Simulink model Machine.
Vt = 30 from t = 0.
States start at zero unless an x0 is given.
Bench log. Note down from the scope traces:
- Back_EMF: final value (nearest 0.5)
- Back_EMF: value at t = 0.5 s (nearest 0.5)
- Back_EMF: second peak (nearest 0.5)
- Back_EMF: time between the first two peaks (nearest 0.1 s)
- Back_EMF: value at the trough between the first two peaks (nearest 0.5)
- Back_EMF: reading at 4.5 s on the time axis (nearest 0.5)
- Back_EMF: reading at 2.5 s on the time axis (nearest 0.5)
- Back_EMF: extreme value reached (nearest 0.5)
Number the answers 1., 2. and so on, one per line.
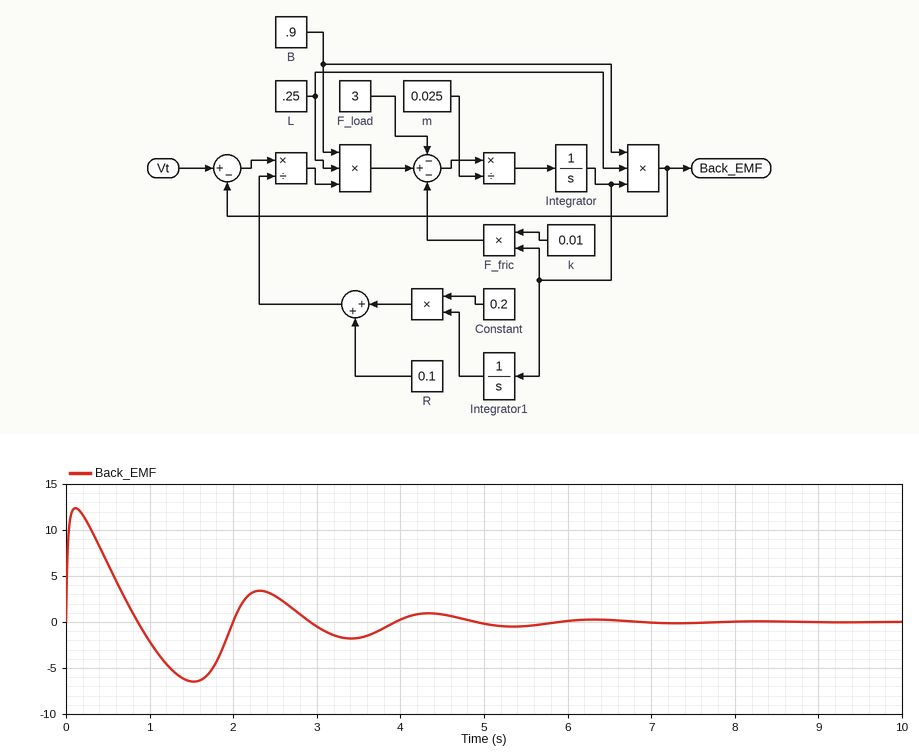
1. 0.0
2. 6.5
3. 3.5
4. 2.2 s
5. -6.5
6. 1.0
7. 3.0
8. 12.5
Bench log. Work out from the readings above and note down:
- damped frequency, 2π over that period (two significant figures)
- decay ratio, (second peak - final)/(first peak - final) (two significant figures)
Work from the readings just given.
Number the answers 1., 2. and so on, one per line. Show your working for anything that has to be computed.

1. 2π / 2.2 = 2.9 rad/s
2. (3.5 - 0) / (12.5 - 0) = 0.28
